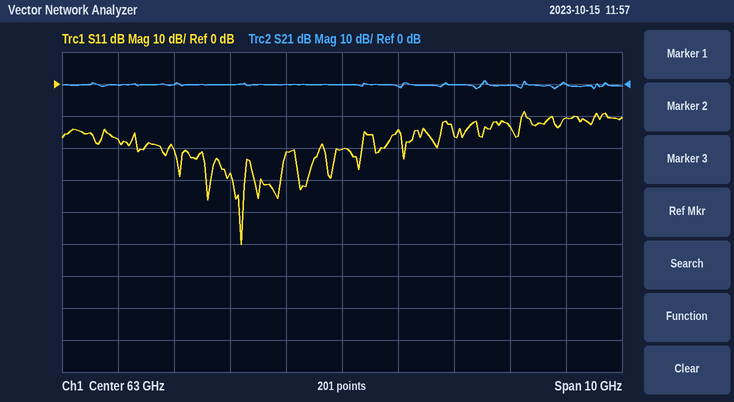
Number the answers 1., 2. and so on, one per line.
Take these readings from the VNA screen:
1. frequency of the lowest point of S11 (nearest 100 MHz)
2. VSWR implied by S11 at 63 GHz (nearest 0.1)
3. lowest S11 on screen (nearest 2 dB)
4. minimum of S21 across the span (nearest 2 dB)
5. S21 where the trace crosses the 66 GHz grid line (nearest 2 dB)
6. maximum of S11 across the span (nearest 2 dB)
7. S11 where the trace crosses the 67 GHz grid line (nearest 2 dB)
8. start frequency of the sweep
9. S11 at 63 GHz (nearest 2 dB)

1. 61.2 GHz
2. 1.2
3. -50 dB
4. -2 dB
5. 0 dB
6. -8 dB
7. -10 dB
8. 58 GHz
9. -20 dB
